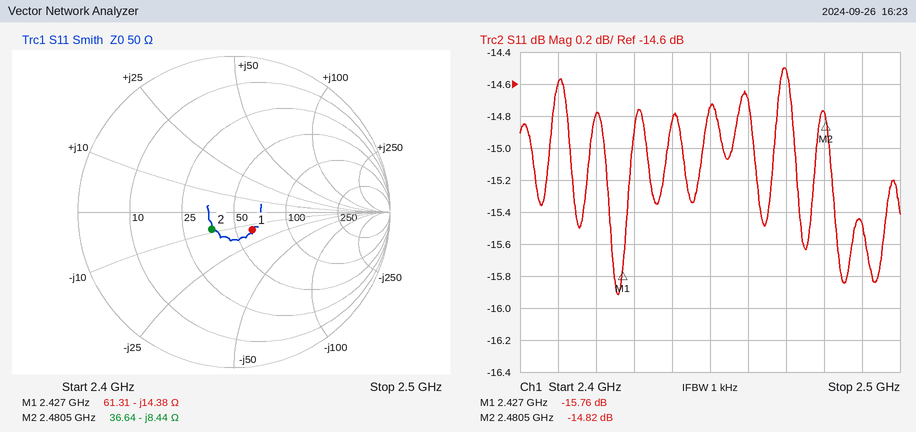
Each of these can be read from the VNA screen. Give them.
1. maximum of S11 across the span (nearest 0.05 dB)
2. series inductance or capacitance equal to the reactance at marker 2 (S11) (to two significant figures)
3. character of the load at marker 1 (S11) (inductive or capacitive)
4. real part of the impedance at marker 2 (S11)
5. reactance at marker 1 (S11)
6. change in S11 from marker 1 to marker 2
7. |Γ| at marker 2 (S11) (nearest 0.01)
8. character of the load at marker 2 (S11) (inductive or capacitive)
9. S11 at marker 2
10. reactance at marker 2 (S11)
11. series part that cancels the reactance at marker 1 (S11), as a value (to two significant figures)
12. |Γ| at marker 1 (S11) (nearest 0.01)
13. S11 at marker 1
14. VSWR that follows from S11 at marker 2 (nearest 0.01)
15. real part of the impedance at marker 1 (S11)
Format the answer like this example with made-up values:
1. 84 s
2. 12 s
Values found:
1. -14.50 dB
2. 7.6 pF
3. capacitive
4. 36.64 Ω
5. -14.38 Ω
6. 0.94 dB
7. 0.18
8. capacitive
9. -14.82 dB
10. -8.44 Ω
11. 940 pH
12. 0.16
13. -15.76 dB
14. 1.44
15. 61.31 Ω
